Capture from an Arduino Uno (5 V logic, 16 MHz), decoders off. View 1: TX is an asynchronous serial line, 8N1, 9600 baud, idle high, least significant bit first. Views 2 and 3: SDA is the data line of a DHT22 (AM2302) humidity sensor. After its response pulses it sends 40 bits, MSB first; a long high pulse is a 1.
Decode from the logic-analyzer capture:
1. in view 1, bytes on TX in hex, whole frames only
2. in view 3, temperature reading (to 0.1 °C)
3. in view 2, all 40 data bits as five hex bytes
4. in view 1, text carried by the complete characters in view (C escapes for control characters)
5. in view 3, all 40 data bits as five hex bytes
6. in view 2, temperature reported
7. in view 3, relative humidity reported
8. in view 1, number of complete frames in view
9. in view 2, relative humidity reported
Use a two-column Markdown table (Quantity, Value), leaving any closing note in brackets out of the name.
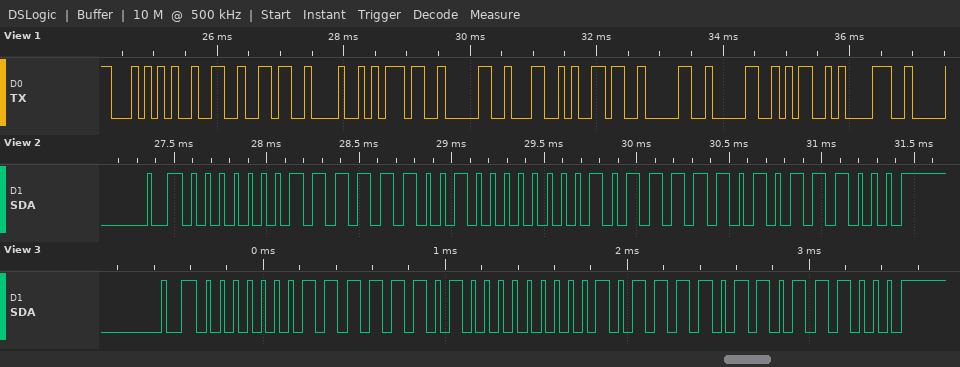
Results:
| Quantity | Value |
|---|---|
| in view 1, bytes on TX in hex, whole frames only | 54 32 36 48 37 30 4C 36 30 30 4D 38 |
| in view 3, temperature reading | 18.9 °C |
| in view 2, all 40 data bits as five hex bytes | 01 F9 00 BE B8 |
| in view 1, text carried by the complete characters in view | "T26H70L600M8" |
| in view 3, all 40 data bits as five hex bytes | 01 FA 00 BD B8 |
| in view 2, temperature reported | 19.0 °C |
| in view 3, relative humidity reported | 50.6 % |
| in view 1, number of complete frames in view | 12 |
| in view 2, relative humidity reported | 50.5 % |
